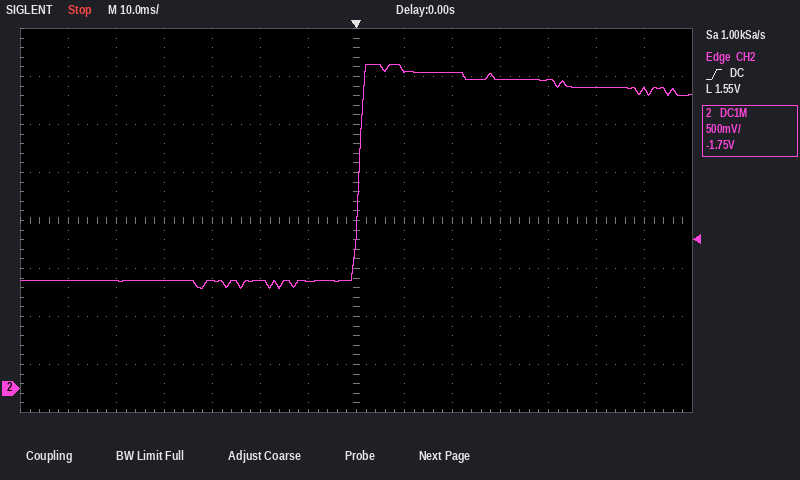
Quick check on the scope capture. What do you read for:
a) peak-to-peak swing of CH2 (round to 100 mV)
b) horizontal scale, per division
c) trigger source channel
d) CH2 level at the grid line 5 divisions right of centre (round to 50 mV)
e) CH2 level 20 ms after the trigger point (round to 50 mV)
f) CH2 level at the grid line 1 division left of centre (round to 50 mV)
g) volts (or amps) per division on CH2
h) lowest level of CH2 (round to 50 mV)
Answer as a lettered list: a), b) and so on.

a) 2.30 V
b) 10 ms
c) CH2
d) 3.15 V
e) 3.30 V
f) 1.10 V
g) 500 mV
h) 1.05 V
